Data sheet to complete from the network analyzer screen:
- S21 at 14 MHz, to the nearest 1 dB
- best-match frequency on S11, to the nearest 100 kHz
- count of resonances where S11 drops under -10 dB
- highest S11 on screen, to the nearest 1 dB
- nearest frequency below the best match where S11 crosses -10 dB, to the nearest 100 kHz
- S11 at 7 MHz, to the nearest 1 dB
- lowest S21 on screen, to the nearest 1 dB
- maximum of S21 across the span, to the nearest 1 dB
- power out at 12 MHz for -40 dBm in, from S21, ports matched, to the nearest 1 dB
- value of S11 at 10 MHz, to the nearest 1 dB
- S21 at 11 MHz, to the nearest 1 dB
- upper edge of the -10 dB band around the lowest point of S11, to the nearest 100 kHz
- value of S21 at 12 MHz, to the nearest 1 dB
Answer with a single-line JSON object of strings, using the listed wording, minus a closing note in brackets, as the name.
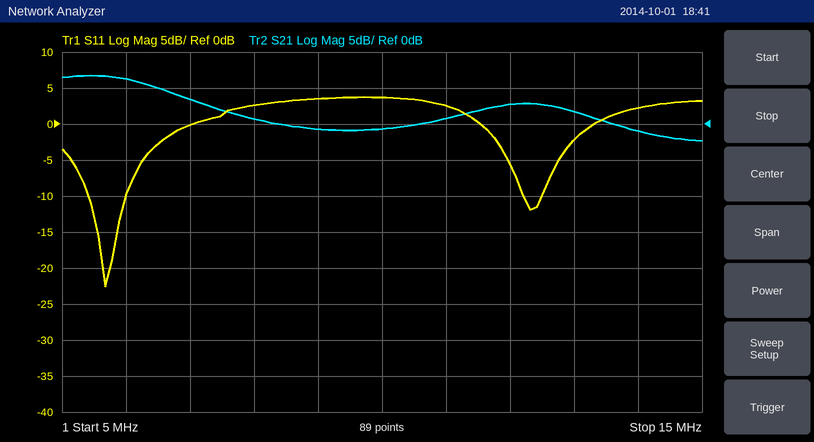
{"S21 at 14 MHz, to the nearest 1 dB": "-1 dB", "best-match frequency on S11, to the nearest 100 kHz": "5.7 MHz", "count of resonances where S11 drops under -10 dB": "2", "highest S11 on screen, to the nearest 1 dB": "4 dB", "nearest frequency below the best match where S11 crosses -10 dB, to the nearest 100 kHz": "5.4 MHz", "S11 at 7 MHz, to the nearest 1 dB": "0 dB", "lowest S21 on screen, to the nearest 1 dB": "-2 dB", "maximum of S21 across the span, to the nearest 1 dB": "7 dB", "power out at 12 MHz for -40 dBm in, from S21, ports matched, to the nearest 1 dB": "-37 dBm", "value of S11 at 10 MHz, to the nearest 1 dB": "4 dB", "S21 at 11 MHz, to the nearest 1 dB": "1 dB", "upper edge of the -10 dB band around the lowest point of S11, to the nearest 100 kHz": "6.0 MHz", "value of S21 at 12 MHz, to the nearest 1 dB": "3 dB"}
